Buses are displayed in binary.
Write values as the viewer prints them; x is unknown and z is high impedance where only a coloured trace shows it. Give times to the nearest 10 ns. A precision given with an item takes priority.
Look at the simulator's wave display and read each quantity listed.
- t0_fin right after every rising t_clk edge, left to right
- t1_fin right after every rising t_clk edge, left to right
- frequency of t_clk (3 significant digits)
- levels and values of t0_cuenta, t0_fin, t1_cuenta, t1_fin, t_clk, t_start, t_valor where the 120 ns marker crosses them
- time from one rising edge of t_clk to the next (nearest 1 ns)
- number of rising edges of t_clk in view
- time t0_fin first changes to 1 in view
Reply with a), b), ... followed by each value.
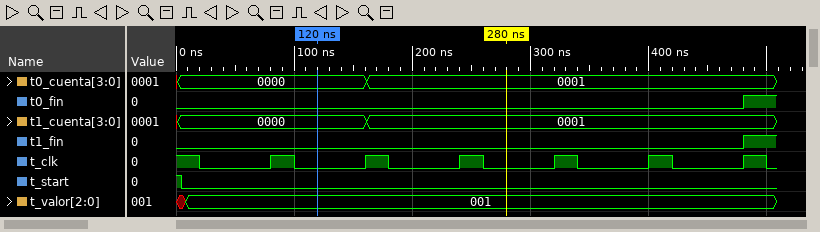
a) 0 0 0 0 0 1
b) 0 0 0 0 0 1
c) 12.5 MHz
d) t0_cuenta=0000, t0_fin=0, t1_cuenta=0000, t1_fin=0, t_clk=0, t_start=0, t_valor=001
e) 80 ns
f) 6
g) 480 ns
